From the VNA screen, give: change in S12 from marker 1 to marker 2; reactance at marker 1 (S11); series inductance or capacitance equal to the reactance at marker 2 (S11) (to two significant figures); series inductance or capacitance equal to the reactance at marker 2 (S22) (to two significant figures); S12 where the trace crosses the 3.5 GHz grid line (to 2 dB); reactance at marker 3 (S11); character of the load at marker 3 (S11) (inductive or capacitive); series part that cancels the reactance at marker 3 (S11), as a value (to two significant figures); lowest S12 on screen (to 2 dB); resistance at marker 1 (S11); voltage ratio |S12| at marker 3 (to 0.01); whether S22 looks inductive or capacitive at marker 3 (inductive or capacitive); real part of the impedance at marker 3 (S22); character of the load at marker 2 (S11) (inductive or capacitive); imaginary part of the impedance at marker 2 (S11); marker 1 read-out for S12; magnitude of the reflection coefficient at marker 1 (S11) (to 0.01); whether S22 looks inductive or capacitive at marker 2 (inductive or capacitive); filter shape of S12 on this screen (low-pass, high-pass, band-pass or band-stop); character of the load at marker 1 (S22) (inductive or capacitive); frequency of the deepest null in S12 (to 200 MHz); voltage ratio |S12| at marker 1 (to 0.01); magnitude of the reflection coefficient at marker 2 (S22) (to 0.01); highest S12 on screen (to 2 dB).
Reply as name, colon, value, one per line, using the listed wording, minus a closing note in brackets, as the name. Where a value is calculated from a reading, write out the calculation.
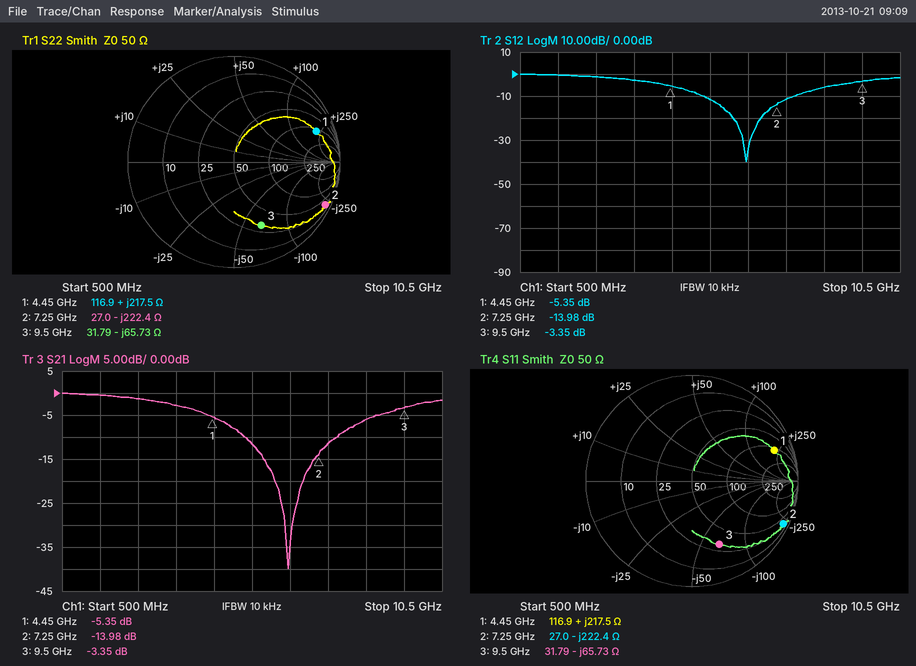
change in S12 from marker 1 to marker 2: -13.98 − (-5.35) = -8.63 dB
reactance at marker 1: +217.5 Ω
series inductance or capacitance equal to the reactance at marker 2 (S11): C = 1/(2π × 7.25 GHz × 222.4 Ω) ≈ 99 fF
series inductance or capacitance equal to the reactance at marker 2 (S22): C = 1/(2π × 7.25 GHz × 222.4 Ω) ≈ 99 fF
S12 where the trace crosses the 3.5 GHz grid line: -2 dB
reactance at marker 3: -65.73 Ω
character of the load at marker 3 (S11): capacitive
series part that cancels the reactance at marker 3 (S11), as a value: L = 65.73 Ω/(2π × 9.5 GHz) ≈ 1.1 nH
lowest S12 on screen: -40 dB
resistance at marker 1: 116.9 Ω
voltage ratio |S12| at marker 3: 10^(-3.35/20) ≈ 0.68
whether S22 looks inductive or capacitive at marker 3: capacitive
real part of the impedance at marker 3: 31.79 Ω
character of the load at marker 2 (S11): capacitive
imaginary part of the impedance at marker 2: -222.4 Ω
marker 1 read-out for S12: -5.35 dB
magnitude of the reflection coefficient at marker 1 (S11): 0.83
whether S22 looks inductive or capacitive at marker 2: capacitive
filter shape of S12 on this screen: band-stop
character of the load at marker 1 (S22): inductive
frequency of the deepest null in S12: 6.4 GHz
voltage ratio |S12| at marker 1: 10^(-5.35/20) ≈ 0.54
magnitude of the reflection coefficient at marker 2 (S22): 0.95
highest S12 on screen: 0 dB
